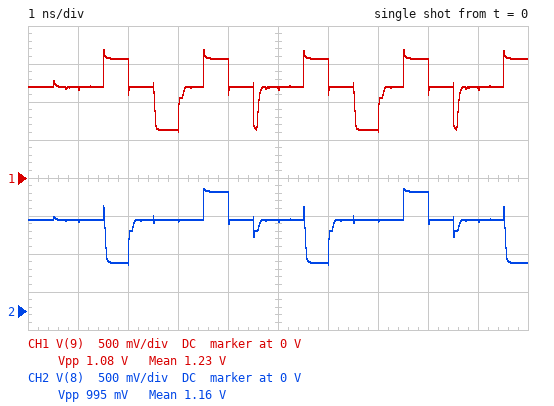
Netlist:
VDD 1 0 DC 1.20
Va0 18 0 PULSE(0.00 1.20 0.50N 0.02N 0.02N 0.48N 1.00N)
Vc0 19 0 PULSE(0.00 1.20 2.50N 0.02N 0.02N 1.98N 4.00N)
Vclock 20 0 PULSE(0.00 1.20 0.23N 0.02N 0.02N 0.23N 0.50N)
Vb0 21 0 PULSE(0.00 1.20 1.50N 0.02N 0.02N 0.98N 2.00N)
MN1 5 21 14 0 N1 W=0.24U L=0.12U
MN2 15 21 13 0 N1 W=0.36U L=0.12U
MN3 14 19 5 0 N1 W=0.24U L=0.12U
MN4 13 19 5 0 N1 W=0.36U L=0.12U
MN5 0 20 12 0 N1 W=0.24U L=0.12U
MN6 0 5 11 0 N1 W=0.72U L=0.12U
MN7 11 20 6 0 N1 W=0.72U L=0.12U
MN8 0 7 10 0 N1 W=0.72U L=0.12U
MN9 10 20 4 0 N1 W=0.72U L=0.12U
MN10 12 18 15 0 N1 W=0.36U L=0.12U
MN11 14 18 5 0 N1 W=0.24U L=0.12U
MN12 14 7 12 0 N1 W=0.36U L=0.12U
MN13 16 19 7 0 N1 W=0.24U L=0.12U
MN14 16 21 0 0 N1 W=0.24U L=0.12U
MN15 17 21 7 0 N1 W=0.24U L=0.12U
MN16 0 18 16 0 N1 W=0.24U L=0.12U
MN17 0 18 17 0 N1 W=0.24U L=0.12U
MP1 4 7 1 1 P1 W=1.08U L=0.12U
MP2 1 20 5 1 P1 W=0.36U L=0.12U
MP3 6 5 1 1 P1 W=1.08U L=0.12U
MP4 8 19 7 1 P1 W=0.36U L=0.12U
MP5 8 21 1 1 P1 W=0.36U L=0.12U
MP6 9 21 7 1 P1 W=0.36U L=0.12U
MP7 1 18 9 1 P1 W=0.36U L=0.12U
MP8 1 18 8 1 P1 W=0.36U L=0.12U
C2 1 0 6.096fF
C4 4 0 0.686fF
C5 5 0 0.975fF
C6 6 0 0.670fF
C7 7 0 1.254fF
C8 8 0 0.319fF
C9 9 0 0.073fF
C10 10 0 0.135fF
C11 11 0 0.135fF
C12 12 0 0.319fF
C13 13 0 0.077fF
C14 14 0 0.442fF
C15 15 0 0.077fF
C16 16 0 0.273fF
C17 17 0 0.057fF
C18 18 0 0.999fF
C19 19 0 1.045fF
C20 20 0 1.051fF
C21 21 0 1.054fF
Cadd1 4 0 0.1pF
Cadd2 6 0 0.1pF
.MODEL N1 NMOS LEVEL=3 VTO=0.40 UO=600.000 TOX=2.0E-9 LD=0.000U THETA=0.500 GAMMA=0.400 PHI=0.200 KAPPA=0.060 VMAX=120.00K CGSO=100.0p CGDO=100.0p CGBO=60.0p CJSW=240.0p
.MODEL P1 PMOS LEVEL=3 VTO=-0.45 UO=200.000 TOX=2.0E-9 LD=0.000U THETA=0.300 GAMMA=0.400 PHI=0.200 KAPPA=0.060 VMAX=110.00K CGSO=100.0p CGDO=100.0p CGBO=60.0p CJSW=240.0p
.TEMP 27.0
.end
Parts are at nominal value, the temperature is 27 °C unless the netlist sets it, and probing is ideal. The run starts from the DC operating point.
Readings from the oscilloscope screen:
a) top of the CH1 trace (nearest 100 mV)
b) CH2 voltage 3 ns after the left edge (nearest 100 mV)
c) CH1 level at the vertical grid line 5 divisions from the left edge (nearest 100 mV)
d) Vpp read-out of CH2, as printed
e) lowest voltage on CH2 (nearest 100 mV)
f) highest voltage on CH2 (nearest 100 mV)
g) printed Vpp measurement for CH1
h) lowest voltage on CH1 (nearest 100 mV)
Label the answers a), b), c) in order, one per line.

a) 1.7 V
b) 1.2 V
c) 1.2 V
d) 995 mV
e) 600 mV
f) 1.6 V
g) 1.08 V
h) 600 mV
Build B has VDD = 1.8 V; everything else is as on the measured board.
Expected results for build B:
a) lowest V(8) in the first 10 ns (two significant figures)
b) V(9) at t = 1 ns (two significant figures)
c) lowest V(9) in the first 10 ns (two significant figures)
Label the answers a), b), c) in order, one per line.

a) 900 mV
b) 1.8 V
c) 840 mV
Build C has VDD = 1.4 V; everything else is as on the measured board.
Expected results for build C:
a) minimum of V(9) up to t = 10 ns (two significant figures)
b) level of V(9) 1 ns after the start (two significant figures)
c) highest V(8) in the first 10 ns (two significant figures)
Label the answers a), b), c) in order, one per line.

a) 650 mV
b) 1.4 V
c) 1.7 V
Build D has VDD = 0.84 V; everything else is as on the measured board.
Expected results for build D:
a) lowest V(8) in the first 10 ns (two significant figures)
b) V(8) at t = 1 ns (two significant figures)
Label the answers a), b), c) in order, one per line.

a) 520 mV
b) 840 mV
